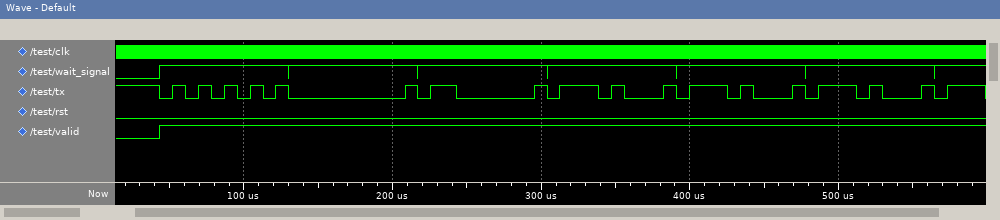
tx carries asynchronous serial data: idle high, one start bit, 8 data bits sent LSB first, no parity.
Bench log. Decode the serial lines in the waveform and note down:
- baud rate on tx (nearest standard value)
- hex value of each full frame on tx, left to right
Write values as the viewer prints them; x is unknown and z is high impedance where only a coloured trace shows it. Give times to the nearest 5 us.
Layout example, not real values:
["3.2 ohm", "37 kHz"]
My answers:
["115200 baud", "55, 00, 03, 17, 17, 17"]
